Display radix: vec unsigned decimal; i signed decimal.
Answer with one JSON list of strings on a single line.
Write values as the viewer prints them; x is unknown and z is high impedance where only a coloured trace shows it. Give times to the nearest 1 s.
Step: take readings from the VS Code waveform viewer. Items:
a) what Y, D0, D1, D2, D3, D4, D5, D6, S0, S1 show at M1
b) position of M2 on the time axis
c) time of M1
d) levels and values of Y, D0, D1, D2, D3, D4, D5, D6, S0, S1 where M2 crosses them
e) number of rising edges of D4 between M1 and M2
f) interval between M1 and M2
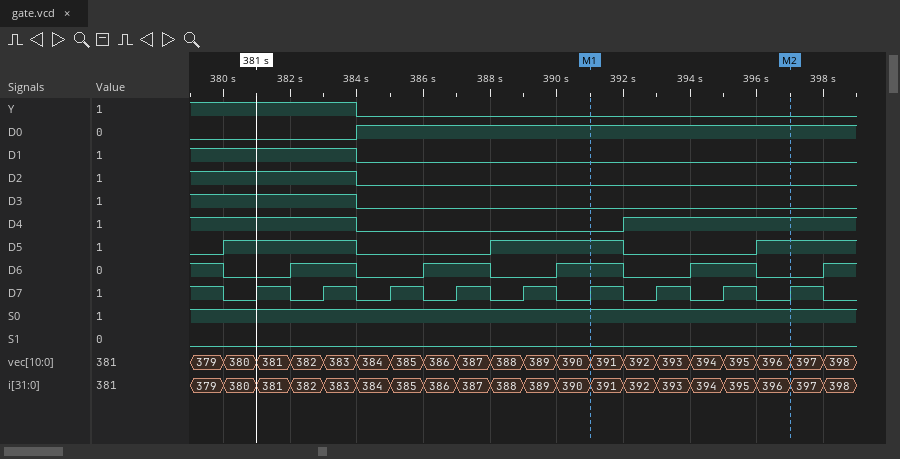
["Y=0, D0=1, D1=0, D2=0, D3=0, D4=0, D5=1, D6=1, S0=1, S1=0", "397 s", "391 s", "Y=0, D0=1, D1=0, D2=0, D3=0, D4=1, D5=1, D6=0, S0=1, S1=0", "1", "6 s"]
